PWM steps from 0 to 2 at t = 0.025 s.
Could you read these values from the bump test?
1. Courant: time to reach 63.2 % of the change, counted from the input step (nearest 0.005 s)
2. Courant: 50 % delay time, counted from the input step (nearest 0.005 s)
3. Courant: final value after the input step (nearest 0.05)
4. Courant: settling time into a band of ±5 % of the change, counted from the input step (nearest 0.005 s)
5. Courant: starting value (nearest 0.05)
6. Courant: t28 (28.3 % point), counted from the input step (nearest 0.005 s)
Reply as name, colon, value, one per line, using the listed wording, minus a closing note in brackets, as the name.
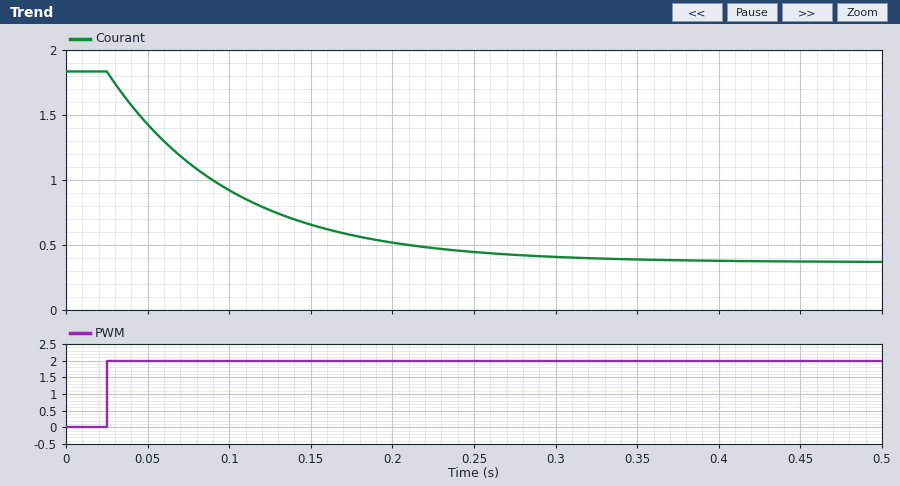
Courant: time to reach 63.2 % of the change, counted from the input step: 0.075 s
Courant: 50 % delay time, counted from the input step: 0.055 s
Courant: final value after the input step: 0.35
Courant: settling time into a band of ±5 % of the change, counted from the input step: 0.230 s
Courant: starting value: 1.85
Courant: t28 (28.3 % point), counted from the input step: 0.025 s
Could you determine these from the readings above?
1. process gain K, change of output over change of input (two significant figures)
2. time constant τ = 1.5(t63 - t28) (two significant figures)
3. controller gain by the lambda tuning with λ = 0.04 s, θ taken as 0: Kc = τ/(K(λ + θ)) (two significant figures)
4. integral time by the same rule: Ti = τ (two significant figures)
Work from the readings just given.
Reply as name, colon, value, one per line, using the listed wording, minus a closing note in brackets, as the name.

process gain K, change of output over change of input: -0.75
time constant τ = 1.5(t63 - t28): 0.075 s
controller gain by the lambda tuning with λ = 0.04 s, θ taken as 0: Kc = τ/(K(λ + θ)): -2.5
integral time by the same rule: Ti = τ: 0.075 s
